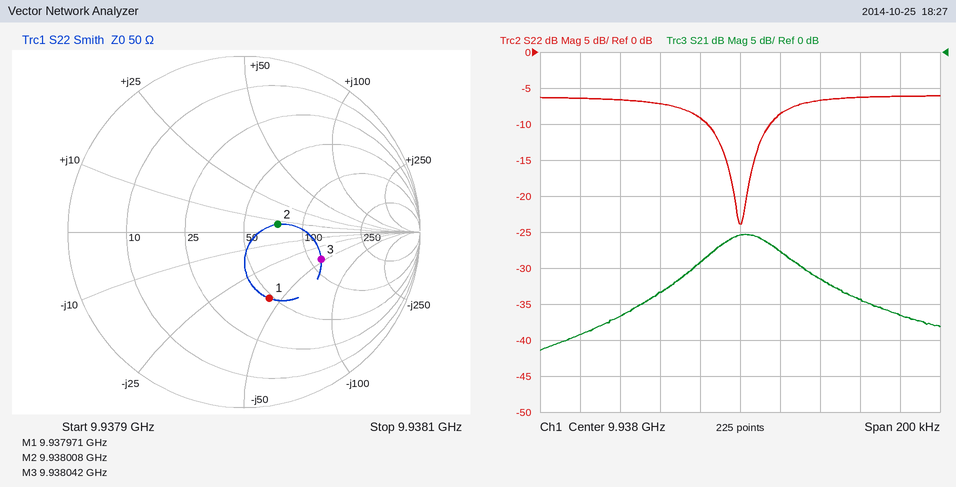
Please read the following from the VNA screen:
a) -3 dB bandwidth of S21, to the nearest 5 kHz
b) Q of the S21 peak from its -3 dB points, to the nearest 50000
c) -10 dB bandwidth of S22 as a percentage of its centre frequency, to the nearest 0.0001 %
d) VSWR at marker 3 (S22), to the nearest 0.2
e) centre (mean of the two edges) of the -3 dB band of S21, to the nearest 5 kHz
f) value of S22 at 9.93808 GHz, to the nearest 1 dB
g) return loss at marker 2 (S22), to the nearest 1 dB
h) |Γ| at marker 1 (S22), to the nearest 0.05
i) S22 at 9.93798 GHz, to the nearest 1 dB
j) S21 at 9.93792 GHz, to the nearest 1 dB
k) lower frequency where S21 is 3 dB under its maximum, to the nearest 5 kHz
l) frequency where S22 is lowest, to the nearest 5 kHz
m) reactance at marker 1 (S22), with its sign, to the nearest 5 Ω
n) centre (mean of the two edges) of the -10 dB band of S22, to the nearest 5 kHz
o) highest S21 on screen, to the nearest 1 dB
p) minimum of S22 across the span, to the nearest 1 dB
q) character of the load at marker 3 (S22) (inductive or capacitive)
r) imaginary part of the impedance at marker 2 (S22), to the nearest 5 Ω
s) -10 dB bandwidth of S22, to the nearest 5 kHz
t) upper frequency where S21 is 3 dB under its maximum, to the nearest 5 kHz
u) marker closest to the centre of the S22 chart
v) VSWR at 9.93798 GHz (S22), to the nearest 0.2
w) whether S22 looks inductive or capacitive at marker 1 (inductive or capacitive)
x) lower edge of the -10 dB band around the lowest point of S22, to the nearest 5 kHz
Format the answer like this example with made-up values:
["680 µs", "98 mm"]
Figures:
["40 kHz", "250000", "0.0003 %", "2.8", "9.938005 GHz", "-6 dB", "14 dB", "0.40", "-9 dB", "-39 dB", "9.937985 GHz", "9.938000 GHz", "-45 Ω", "9.938000 GHz", "-25 dB", "-24 dB", "capacitive", "+5 Ω", "30 kHz", "9.938025 GHz", "marker 2", "2.0", "capacitive", "9.937985 GHz"]
